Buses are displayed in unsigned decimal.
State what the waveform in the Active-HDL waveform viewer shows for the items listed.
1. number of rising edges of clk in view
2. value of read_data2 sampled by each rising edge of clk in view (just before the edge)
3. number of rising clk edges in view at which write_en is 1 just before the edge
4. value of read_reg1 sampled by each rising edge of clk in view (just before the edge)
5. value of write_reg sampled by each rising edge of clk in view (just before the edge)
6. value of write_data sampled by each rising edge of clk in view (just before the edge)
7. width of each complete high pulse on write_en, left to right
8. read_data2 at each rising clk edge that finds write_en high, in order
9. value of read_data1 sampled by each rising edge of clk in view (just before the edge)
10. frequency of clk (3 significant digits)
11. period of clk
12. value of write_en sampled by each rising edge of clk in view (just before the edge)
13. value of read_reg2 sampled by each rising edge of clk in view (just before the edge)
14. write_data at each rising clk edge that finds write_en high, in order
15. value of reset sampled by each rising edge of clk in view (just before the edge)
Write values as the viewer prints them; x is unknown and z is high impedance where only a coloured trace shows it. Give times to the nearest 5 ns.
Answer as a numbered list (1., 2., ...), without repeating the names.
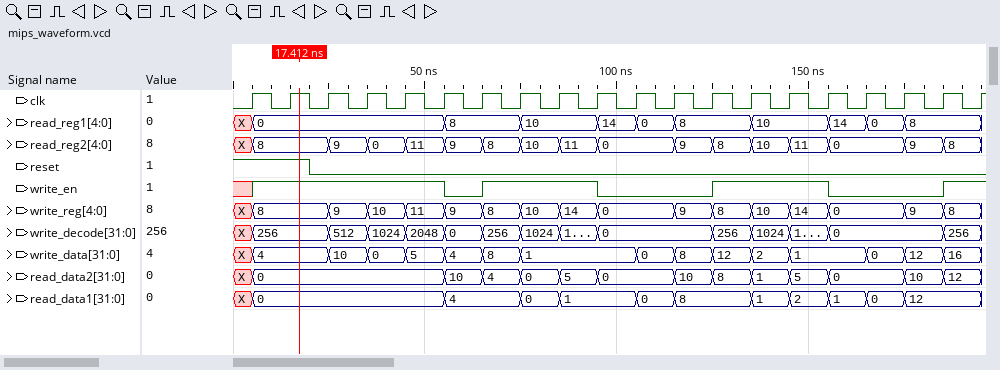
1. 20
2. X, 0, 0, 0, 0, 0, 10, 4, 0, 5, 0, 0, 10, 8, 1, 5, 0, 0, 10, 12
3. 12
4. X, 0, 0, 0, 0, 0, 8, 8, 10, 10, 14, 0, 8, 8, 10, 10, 14, 0, 8, 8
5. X, 8, 8, 9, 10, 11, 9, 8, 10, 14, 0, 0, 9, 8, 10, 14, 0, 0, 9, 8
6. X, 4, 4, 10, 0, 5, 4, 8, 1, 1, 1, 0, 8, 12, 2, 1, 1, 0, 12, 16
7. 30 ns, 30 ns
8. 0, 0, 0, 0, 0, 4, 0, 5, 8, 1, 5, 12
9. X, 0, 0, 0, 0, 0, 4, 4, 0, 1, 1, 0, 8, 8, 1, 2, 1, 0, 12, 12
10. 100 MHz
11. 10 ns
12. x 1 1 1 1 1 0 1 1 1 0 0 0 1 1 1 0 0 0 1
13. X, 8, 8, 9, 0, 11, 9, 8, 10, 11, 0, 0, 9, 8, 10, 11, 0, 0, 9, 8
14. 4, 4, 10, 0, 5, 8, 1, 1, 12, 2, 1, 16
15. 1 1 0 0 0 0 0 0 0 0 0 0 0 0 0 0 0 0 0 0
